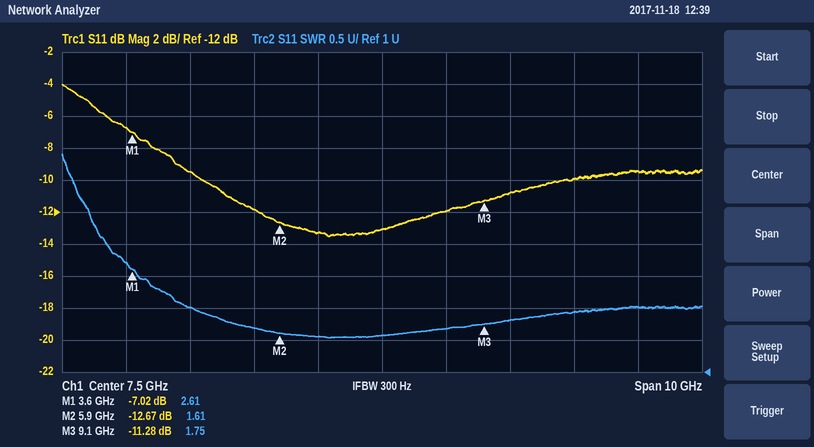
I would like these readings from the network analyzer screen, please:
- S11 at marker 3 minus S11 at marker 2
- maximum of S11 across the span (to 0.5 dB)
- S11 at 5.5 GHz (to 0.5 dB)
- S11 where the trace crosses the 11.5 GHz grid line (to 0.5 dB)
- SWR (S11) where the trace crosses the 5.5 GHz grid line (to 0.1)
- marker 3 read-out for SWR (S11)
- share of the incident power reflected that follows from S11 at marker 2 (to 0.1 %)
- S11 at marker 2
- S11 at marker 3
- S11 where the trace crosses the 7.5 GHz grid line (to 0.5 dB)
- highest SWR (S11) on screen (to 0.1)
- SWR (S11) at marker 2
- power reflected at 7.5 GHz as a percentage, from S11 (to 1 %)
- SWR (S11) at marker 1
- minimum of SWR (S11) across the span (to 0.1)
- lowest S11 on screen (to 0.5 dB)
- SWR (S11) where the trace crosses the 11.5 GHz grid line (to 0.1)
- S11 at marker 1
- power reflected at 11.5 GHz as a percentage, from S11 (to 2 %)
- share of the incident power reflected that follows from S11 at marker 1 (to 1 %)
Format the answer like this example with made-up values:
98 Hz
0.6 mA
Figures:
1.39 dB
-4.0 dB
-12.0 dB
-9.5 dB
1.7
1.75
5.4 %
-12.67 dB
-11.28 dB
-13.0 dB
4.4
1.61
5 %
2.61
1.5
-13.5 dB
2.0
-7.02 dB
12 %
20 %
